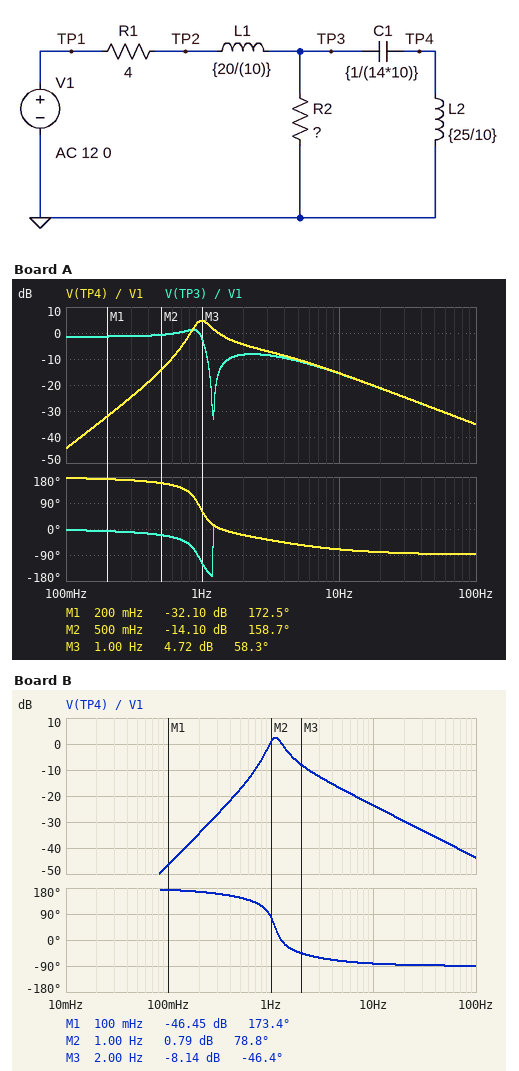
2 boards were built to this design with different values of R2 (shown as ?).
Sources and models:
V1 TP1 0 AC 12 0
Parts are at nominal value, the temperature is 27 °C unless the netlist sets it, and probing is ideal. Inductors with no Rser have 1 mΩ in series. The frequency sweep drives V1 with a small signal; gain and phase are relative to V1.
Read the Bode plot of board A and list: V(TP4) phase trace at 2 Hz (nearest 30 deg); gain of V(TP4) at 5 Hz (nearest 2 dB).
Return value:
-30 deg
-10 dB
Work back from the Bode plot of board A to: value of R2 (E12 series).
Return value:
22 Ω
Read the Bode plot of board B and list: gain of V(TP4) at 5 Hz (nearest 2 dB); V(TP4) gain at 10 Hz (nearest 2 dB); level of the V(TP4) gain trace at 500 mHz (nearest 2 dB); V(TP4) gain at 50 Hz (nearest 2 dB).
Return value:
-18 dB
-24 dB
-18 dB
-38 dB
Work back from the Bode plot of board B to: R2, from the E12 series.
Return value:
8.2 Ω
